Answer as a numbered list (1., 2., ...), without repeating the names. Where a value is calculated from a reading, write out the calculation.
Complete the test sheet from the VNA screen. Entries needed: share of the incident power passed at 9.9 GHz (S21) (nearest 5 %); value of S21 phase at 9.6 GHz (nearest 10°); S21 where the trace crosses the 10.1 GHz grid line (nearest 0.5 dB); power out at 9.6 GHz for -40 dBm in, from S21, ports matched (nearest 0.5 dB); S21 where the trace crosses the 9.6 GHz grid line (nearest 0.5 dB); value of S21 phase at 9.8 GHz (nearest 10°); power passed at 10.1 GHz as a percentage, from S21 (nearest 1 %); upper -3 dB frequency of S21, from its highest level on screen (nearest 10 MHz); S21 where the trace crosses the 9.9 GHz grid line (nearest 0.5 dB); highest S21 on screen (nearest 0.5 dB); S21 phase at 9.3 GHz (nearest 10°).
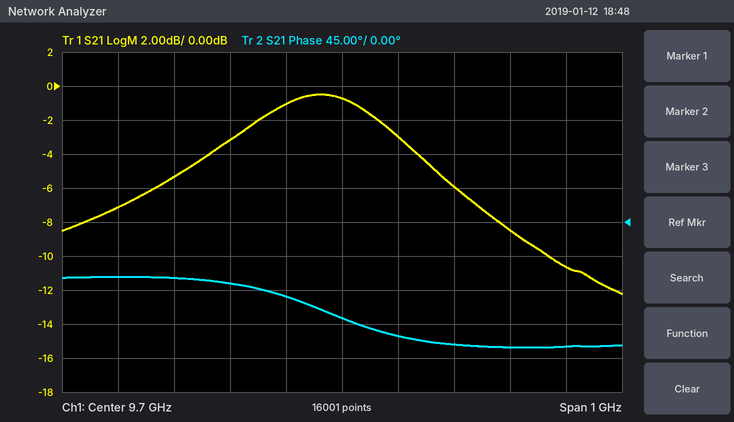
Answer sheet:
1. 10^(-6/10) ≈ 25 %
2. -100°
3. -10.5 dB
4. -40 dBm + (-1.0 dB) = -41.0 dBm
5. -1.0 dB
6. -150°
7. 10^(-10.5/10) ≈ 9 %
8. 9.82 GHz
9. -6.0 dB
10. -0.5 dB
11. -70°
